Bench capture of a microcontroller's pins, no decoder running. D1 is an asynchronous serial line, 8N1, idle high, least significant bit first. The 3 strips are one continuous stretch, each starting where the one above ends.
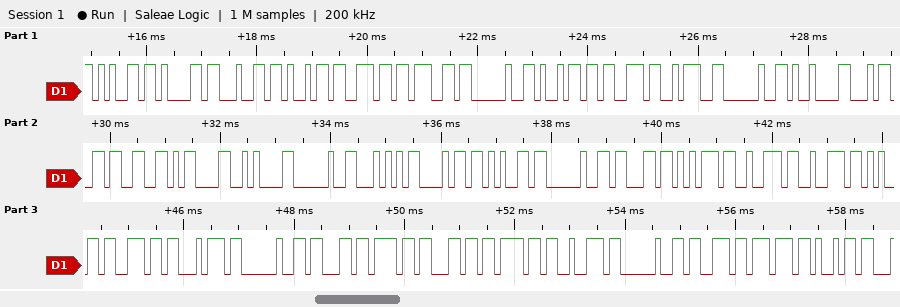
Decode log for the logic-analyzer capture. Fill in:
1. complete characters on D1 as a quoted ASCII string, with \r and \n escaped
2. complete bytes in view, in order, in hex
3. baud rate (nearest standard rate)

"eading is: \t43\r\n The current color swi"
0x65 0x61 0x64 0x69 0x6E 0x67 0x20 0x69 0x73 0x3A 0x20 0x09 0x34 0x33 0x0D 0x0A 0x20 0x54 0x68 0x65 0x20 0x63 0x75 0x72 0x72 0x65 0x6E 0x74 0x20 0x63 0x6F 0x6C 0x6F 0x72 0x20 0x73 0x77 0x69
9600 baud
